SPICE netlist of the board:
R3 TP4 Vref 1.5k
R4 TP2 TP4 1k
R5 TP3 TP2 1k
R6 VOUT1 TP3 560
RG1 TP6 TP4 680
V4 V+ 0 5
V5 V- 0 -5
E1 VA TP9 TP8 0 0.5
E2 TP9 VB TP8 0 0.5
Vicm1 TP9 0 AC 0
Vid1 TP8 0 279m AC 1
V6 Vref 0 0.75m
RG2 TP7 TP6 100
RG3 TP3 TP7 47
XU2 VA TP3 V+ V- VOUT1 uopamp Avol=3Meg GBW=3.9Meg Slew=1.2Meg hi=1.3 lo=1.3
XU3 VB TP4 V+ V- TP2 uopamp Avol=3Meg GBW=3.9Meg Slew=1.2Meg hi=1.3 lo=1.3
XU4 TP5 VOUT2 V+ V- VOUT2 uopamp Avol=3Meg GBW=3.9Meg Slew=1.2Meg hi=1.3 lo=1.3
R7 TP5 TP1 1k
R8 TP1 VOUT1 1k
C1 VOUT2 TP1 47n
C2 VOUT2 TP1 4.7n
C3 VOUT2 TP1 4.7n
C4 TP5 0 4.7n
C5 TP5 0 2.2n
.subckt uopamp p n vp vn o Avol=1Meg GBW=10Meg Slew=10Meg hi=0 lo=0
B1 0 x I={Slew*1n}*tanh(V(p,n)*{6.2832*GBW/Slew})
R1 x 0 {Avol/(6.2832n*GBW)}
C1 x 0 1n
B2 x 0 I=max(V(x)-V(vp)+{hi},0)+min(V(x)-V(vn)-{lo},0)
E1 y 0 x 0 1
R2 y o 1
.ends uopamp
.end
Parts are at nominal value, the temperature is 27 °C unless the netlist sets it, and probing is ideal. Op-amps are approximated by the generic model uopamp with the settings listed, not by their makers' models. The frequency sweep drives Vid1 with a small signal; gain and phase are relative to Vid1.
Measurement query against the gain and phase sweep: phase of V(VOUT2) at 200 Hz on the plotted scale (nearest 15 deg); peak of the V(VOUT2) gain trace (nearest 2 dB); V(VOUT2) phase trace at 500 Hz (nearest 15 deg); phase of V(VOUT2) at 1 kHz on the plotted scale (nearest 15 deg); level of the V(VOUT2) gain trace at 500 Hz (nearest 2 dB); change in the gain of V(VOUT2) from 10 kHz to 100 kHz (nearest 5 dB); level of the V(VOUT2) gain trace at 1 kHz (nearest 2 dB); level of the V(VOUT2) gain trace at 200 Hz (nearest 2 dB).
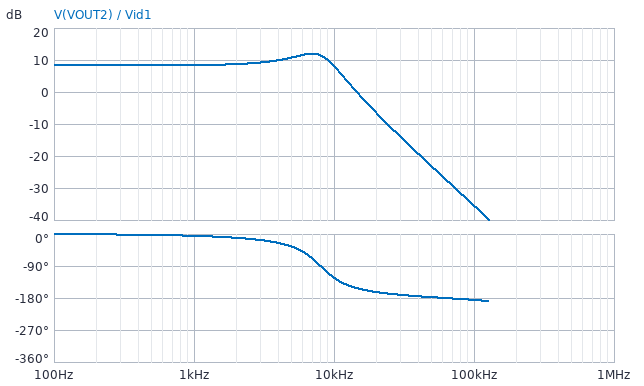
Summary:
0 deg
12 dB
0 deg
0 deg
8 dB
-45 dB
8 dB
8 dB
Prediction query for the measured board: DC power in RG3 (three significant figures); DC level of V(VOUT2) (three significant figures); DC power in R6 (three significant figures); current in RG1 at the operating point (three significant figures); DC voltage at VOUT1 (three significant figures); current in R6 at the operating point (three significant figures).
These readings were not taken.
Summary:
5.35 µW
726 mV
614 µW
337 µA
726 mV
1.05 mA
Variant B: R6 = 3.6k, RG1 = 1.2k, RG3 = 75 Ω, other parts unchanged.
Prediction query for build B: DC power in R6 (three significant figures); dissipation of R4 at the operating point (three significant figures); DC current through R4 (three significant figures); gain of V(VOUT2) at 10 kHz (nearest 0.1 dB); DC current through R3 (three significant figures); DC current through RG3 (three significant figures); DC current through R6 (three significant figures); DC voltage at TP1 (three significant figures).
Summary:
2.18 mW
87.9 µW
296 µA
20.2 dB
93.5 µA
203 µA
778 µA
2.94 V
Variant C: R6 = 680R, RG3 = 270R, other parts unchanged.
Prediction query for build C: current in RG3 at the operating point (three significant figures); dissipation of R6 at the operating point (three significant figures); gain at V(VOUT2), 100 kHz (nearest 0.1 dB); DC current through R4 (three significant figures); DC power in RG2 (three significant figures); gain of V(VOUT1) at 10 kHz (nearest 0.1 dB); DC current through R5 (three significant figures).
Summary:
266 µA
556 µW
-35.2 dB
359 µA
7.06 µW
8.6 dB
638 µA
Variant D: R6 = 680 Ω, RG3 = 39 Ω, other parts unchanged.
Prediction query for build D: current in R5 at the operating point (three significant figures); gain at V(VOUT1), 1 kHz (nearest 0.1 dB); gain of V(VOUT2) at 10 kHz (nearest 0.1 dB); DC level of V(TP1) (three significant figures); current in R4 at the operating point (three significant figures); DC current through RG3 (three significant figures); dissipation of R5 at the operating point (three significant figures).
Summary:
713 µA
9.7 dB
9.5 dB
856 mV
434 µA
341 µA
509 µW
